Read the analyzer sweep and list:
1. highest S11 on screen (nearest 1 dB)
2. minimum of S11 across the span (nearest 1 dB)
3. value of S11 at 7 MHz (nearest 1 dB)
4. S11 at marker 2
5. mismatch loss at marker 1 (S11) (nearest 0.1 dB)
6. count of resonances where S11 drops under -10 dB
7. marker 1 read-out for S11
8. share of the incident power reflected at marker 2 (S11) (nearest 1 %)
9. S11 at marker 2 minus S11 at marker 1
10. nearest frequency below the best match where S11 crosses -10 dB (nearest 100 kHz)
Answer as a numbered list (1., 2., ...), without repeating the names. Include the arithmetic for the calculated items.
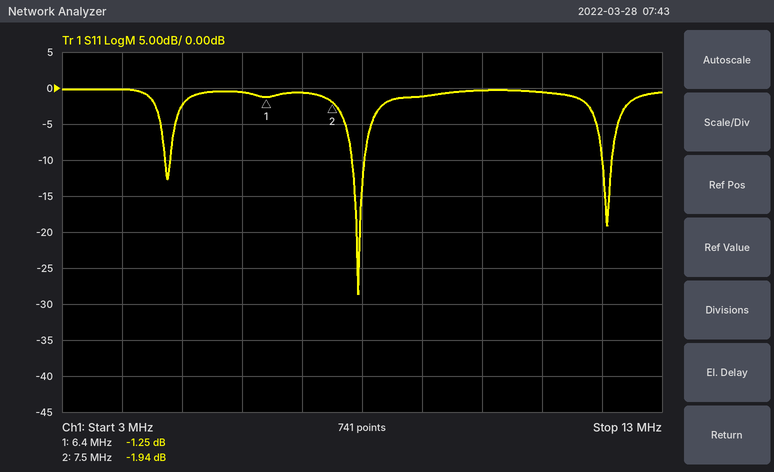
1. 0 dB
2. -29 dB
3. -1 dB
4. -1.94 dB
5. −10 log10(1 − 10^(-1.25/10)) ≈ 6.0 dB
6. 3
7. -1.25 dB
8. 10^(-1.94/10) ≈ 64 %
9. -1.94 − (-1.25) = -0.69 dB
10. 7.8 MHz
